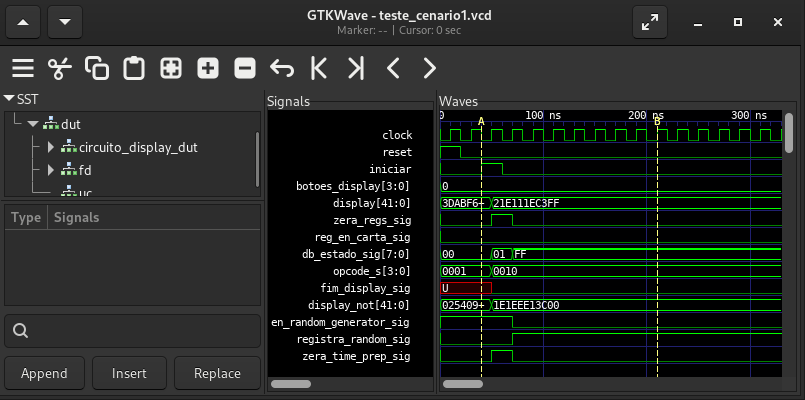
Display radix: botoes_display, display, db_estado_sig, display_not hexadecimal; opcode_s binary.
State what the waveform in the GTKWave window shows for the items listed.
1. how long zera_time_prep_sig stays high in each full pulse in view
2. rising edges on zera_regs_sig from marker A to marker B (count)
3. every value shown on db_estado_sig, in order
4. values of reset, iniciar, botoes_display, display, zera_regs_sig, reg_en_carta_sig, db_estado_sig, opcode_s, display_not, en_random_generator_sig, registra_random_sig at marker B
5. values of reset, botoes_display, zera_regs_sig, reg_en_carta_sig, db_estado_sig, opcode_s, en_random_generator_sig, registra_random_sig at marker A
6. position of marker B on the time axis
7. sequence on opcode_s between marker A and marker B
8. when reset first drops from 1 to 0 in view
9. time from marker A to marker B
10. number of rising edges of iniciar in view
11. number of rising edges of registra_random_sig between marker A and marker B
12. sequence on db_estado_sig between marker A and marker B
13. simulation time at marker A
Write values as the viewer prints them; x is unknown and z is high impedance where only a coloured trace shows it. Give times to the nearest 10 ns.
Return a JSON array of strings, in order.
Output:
["20 ns", "1", "00, 01, FF", "reset=0, iniciar=0, botoes_display=0, display=21E111EC3FF, zera_regs_sig=0, reg_en_carta_sig=0, db_estado_sig=FF, opcode_s=0010, display_not=1E1EEE13C00, en_random_generator_sig=0, registra_random_sig=1", "reset=0, botoes_display=0, zera_regs_sig=0, reg_en_carta_sig=0, db_estado_sig=00, opcode_s=0001, en_random_generator_sig=1, registra_random_sig=0", "210 ns", "0001, 0010", "20 ns", "170 ns", "1", "1", "00, 01, FF", "40 ns"]
